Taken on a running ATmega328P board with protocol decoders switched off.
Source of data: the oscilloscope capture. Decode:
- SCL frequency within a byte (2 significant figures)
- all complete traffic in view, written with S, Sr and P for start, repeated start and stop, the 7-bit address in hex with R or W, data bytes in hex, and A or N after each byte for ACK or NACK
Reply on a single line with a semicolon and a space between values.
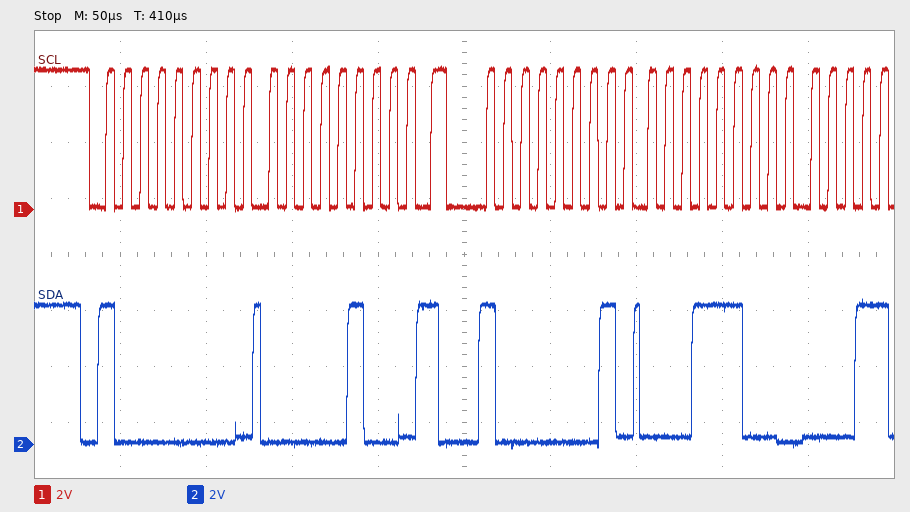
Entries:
100 kHz; S 40W A 04 A Sr 40R A 1C A
